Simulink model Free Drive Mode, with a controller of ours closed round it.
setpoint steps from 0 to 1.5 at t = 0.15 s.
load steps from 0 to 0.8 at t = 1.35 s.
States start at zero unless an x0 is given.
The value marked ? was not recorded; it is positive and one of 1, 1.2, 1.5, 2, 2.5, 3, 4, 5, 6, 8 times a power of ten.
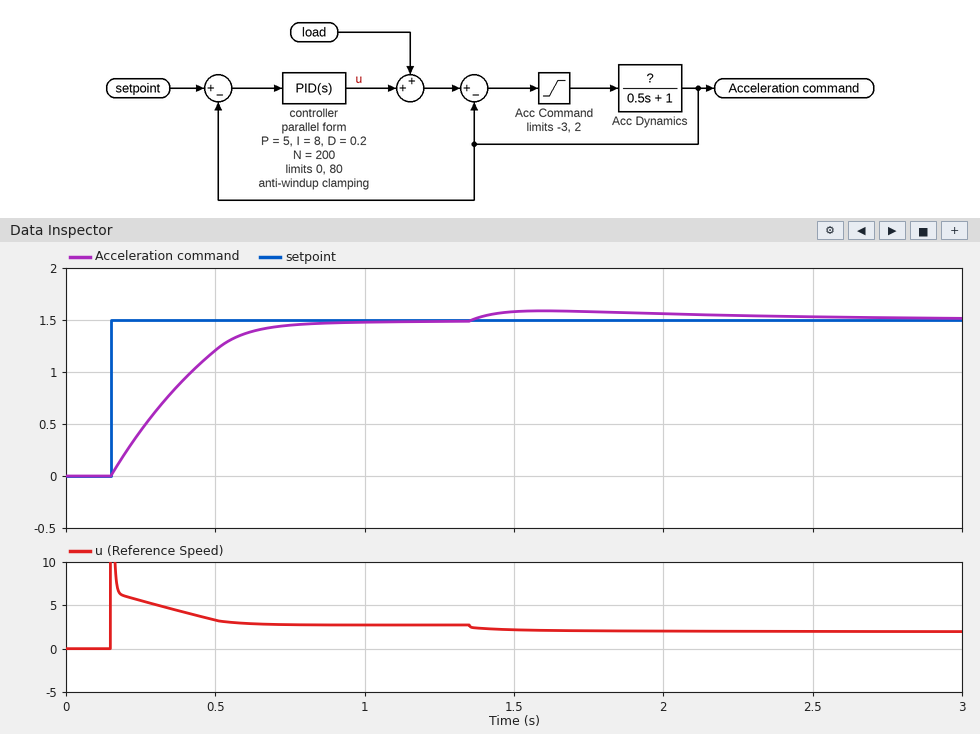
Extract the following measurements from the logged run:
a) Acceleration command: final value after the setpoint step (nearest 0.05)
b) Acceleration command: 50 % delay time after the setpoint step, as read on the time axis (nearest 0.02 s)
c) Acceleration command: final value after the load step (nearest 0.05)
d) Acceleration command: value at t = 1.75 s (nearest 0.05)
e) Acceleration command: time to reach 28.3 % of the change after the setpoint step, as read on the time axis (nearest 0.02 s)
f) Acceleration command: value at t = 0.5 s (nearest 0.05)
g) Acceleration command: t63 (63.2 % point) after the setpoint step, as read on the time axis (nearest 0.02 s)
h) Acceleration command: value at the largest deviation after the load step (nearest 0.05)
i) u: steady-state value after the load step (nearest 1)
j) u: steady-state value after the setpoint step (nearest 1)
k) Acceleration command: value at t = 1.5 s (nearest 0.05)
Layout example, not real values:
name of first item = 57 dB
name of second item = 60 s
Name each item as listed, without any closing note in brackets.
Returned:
Acceleration command: final value after the setpoint step = 1.50
Acceleration command: 50 % delay time after the setpoint step, as read on the time axis = 0.34 s
Acceleration command: final value after the load step = 1.50
Acceleration command: value at t = 1.75 s = 1.60
Acceleration command: time to reach 28.3 % of the change after the setpoint step, as read on the time axis = 0.24 s
Acceleration command: value at t = 0.5 s = 1.20
Acceleration command: t63 (63.2 % point) after the setpoint step, as read on the time axis = 0.40 s
Acceleration command: value at the largest deviation after the load step = 1.60
u: steady-state value after the load step = 2
u: steady-state value after the setpoint step = 3
Acceleration command: value at t = 1.5 s = 1.60
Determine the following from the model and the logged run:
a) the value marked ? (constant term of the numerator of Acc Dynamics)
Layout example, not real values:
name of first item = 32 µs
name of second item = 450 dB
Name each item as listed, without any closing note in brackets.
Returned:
the value marked ? = 1.2
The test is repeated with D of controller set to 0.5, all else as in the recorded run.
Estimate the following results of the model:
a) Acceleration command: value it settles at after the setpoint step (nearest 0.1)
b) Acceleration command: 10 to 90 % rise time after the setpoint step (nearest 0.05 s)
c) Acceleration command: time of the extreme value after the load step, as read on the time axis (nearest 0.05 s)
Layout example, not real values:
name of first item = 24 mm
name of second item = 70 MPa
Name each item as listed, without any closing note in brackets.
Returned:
Acceleration command: value it settles at after the setpoint step = 1.5
Acceleration command: 10 to 90 % rise time after the setpoint step = 0.45 s
Acceleration command: time of the extreme value after the load step, as read on the time axis = 1.65 s
